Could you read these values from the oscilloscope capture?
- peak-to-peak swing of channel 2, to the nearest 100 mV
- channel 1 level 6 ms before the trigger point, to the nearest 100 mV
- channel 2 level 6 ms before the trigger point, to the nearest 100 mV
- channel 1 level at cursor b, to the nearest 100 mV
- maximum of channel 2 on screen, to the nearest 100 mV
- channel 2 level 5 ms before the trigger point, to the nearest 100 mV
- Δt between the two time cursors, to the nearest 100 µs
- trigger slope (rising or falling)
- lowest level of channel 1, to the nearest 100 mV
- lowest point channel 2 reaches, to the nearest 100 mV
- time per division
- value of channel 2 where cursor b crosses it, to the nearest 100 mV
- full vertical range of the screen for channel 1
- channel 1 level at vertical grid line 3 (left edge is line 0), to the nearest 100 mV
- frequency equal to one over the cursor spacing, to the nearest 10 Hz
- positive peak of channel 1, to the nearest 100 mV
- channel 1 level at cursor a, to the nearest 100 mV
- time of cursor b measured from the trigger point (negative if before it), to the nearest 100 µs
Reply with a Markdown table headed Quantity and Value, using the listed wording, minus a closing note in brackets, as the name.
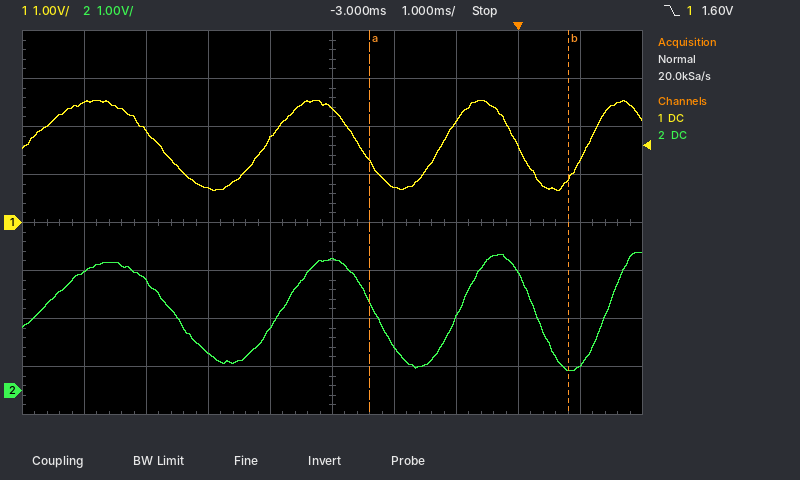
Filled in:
| Quantity | Value |
|---|---|
| peak-to-peak swing of channel 2, to the nearest 100 mV | 2.5 V |
| channel 1 level 6 ms before the trigger point, to the nearest 100 mV | 1.9 V |
| channel 2 level 6 ms before the trigger point, to the nearest 100 mV | 2.3 V |
| channel 1 level at cursor b, to the nearest 100 mV | 900 mV |
| maximum of channel 2 on screen, to the nearest 100 mV | 2.9 V |
| channel 2 level 5 ms before the trigger point, to the nearest 100 mV | 800 mV |
| Δt between the two time cursors, to the nearest 100 µs | 3.2 ms |
| trigger slope | falling |
| lowest level of channel 1, to the nearest 100 mV | 700 mV |
| lowest point channel 2 reaches, to the nearest 100 mV | 400 mV |
| time per division | 1 ms |
| value of channel 2 where cursor b crosses it, to the nearest 100 mV | 400 mV |
| full vertical range of the screen for channel 1 | 8 V |
| channel 1 level at vertical grid line 3 (left edge is line 0), to the nearest 100 mV | 700 mV |
| frequency equal to one over the cursor spacing, to the nearest 10 Hz | 310 Hz |
| positive peak of channel 1, to the nearest 100 mV | 2.5 V |
| channel 1 level at cursor a, to the nearest 100 mV | 1.3 V |
| time of cursor b measured from the trigger point (negative if before it), to the nearest 100 µs | +800 µs |
